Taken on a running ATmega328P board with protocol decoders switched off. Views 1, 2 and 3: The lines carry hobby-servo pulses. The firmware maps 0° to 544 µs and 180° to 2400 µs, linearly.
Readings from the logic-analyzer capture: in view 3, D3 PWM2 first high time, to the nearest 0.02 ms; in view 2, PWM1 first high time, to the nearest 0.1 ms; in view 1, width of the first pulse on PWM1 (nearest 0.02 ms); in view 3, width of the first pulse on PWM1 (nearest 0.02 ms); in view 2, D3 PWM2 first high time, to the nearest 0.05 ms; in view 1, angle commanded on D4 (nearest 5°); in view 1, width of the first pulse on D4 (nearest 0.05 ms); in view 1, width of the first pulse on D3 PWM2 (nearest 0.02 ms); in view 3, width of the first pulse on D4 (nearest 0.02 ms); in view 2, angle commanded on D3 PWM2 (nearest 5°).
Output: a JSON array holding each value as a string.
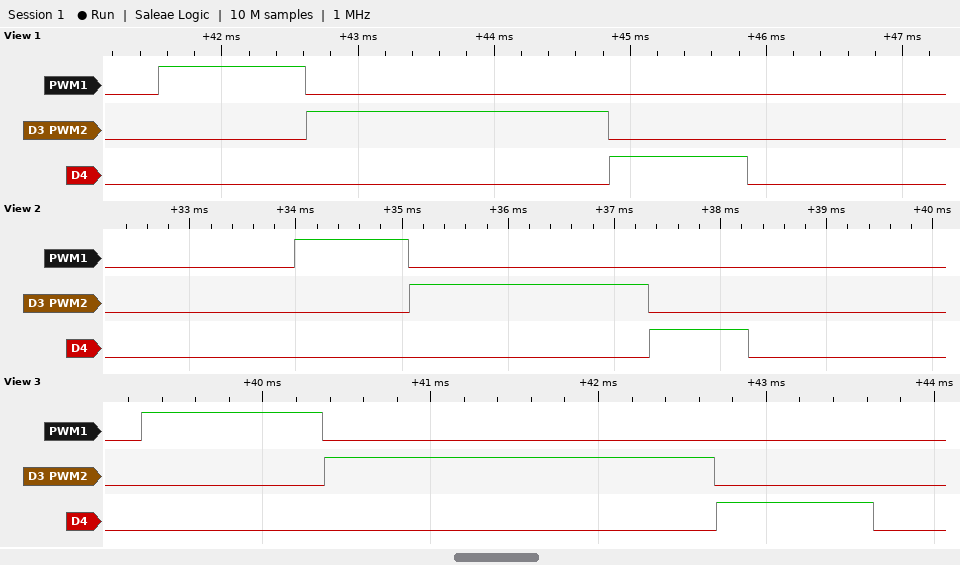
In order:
["2.32 ms", "1.1 ms", "1.08 ms", "1.08 ms", "2.25 ms", "45°", "1.00 ms", "2.22 ms", "0.94 ms", "165°"]
